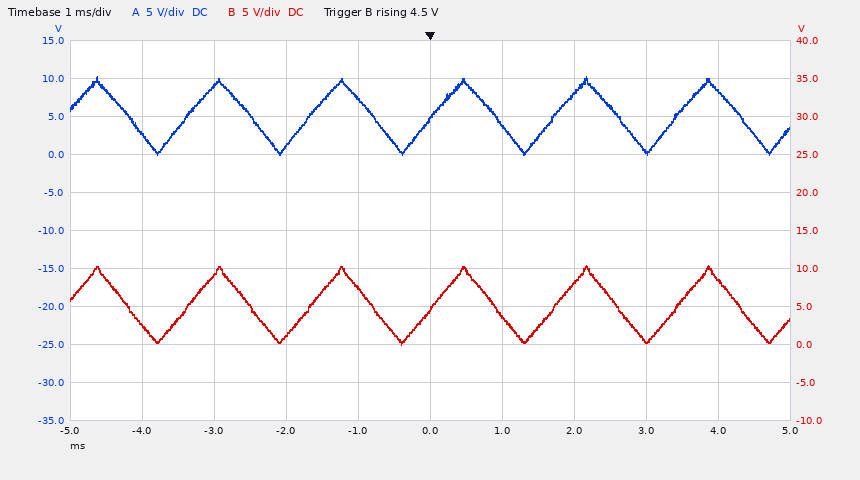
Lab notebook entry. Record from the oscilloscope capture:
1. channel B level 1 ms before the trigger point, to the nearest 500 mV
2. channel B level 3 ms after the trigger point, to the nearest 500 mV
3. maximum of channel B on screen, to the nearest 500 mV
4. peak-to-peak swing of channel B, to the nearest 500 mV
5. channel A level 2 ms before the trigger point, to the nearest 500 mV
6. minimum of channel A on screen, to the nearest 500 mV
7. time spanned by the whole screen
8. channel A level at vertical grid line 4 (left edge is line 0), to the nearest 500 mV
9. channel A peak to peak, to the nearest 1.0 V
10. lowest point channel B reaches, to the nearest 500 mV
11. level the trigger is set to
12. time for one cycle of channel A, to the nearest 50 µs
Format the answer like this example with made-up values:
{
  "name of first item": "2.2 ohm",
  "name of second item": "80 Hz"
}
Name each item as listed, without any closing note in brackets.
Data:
{
  "channel B level 1 ms before the trigger point, to the nearest 500 mV": "7.5 V",
  "channel B level 3 ms after the trigger point, to the nearest 500 mV": "500 mV",
  "maximum of channel B on screen, to the nearest 500 mV": "10.5 V",
  "peak-to-peak swing of channel B, to the nearest 500 mV": "10.5 V",
  "channel A level 2 ms before the trigger point, to the nearest 500 mV": "1.0 V",
  "minimum of channel A on screen, to the nearest 500 mV": "0.0 V",
  "time spanned by the whole screen": "10 ms",
  "channel A level at vertical grid line 4 (left edge is line 0), to the nearest 500 mV": "7.5 V",
  "channel A peak to peak, to the nearest 1.0 V": "10.0 V",
  "lowest point channel B reaches, to the nearest 500 mV": "0.0 V",
  "level the trigger is set to": "4.5 V",
  "time for one cycle of channel A, to the nearest 50 µs": "1.70 ms"
}
